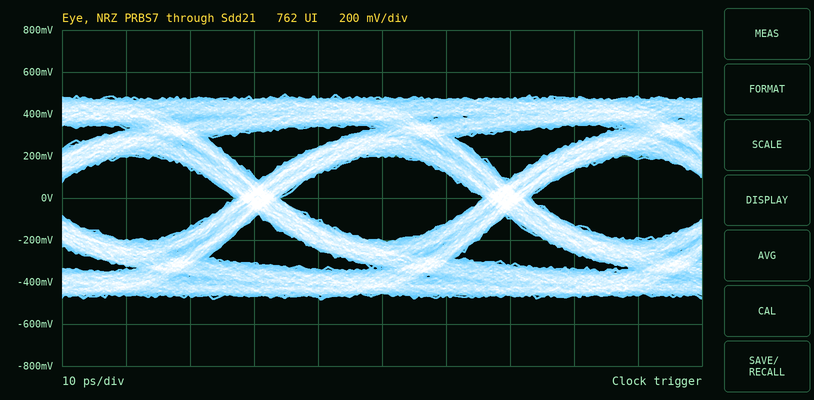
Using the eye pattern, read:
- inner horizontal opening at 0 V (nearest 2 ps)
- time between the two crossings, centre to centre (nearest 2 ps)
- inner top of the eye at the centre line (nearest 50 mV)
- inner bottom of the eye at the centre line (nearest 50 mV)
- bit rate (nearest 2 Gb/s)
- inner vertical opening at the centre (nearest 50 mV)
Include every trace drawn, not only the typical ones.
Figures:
32 ps
38 ps
200 mV
-200 mV
26 Gb/s
400 mV
